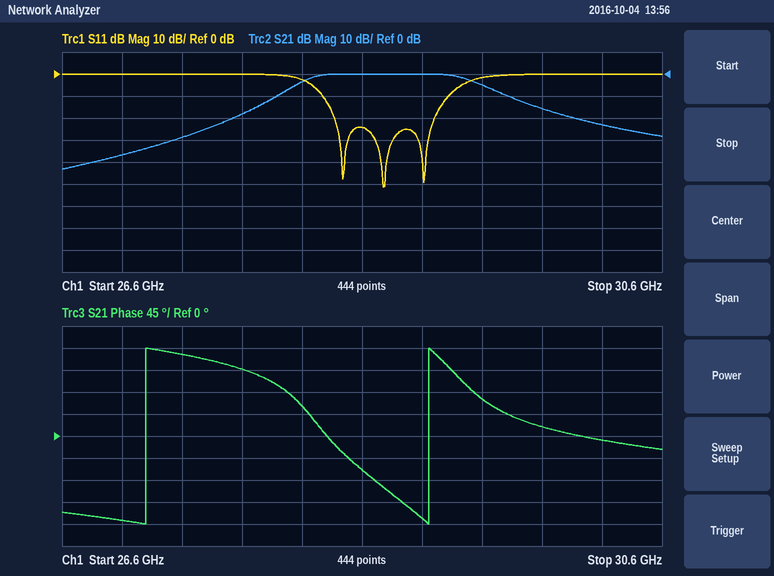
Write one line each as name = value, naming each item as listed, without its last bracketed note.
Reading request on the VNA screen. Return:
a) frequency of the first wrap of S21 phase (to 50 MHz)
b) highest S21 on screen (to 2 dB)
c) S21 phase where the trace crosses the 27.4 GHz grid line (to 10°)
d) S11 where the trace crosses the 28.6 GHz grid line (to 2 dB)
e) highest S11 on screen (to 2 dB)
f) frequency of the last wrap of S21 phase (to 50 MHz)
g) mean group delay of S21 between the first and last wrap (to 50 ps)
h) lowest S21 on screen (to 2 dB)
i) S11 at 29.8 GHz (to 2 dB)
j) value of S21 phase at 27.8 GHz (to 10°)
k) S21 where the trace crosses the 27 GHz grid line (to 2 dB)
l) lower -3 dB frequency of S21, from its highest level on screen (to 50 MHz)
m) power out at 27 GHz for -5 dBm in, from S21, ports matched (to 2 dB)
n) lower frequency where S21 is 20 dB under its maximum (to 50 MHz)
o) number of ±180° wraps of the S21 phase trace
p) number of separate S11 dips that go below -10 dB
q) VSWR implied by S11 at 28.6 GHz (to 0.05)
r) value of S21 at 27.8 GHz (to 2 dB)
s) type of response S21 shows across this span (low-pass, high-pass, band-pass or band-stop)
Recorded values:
frequency of the first wrap of S21 phase = 27.15 GHz
highest S21 on screen = 0 dB
S21 phase where the trace crosses the 27.4 GHz grid line = 170°
S11 where the trace crosses the 28.6 GHz grid line = -24 dB
highest S11 on screen = 0 dB
frequency of the last wrap of S21 phase = 29.05 GHz
mean group delay of S21 between the first and last wrap = 550 ps
lowest S21 on screen = -44 dB
S11 at 29.8 GHz = 0 dB
value of S21 phase at 27.8 GHz = 140°
S21 where the trace crosses the 27 GHz grid line = -36 dB
lower -3 dB frequency of S21, from its highest level on screen = 28.20 GHz
power out at 27 GHz for -5 dBm in, from S21, ports matched = -42 dBm
lower frequency where S21 is 20 dB under its maximum = 27.75 GHz
number of ±180° wraps of the S21 phase trace = 2
number of separate S11 dips that go below -10 dB = 3
VSWR implied by S11 at 28.6 GHz = 1.15
value of S21 at 27.8 GHz = -18 dB
type of response S21 shows across this span = band-pass
